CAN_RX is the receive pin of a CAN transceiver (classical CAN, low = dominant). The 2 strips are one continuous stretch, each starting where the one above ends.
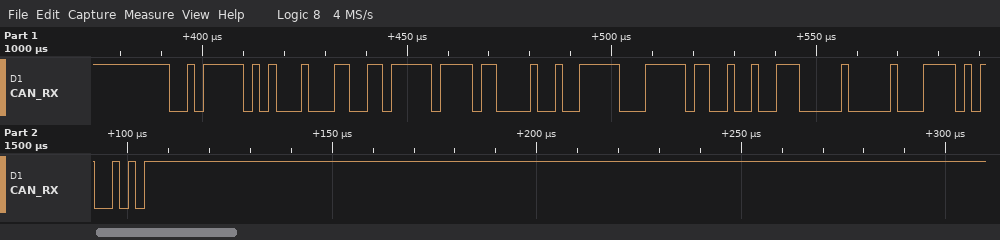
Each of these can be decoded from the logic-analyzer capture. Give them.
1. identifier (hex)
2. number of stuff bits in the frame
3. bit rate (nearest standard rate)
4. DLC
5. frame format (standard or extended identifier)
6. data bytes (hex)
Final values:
0x2FD
6
500 kbit/s
8
standard
CD FF 61 27 CF E4 9C 00
